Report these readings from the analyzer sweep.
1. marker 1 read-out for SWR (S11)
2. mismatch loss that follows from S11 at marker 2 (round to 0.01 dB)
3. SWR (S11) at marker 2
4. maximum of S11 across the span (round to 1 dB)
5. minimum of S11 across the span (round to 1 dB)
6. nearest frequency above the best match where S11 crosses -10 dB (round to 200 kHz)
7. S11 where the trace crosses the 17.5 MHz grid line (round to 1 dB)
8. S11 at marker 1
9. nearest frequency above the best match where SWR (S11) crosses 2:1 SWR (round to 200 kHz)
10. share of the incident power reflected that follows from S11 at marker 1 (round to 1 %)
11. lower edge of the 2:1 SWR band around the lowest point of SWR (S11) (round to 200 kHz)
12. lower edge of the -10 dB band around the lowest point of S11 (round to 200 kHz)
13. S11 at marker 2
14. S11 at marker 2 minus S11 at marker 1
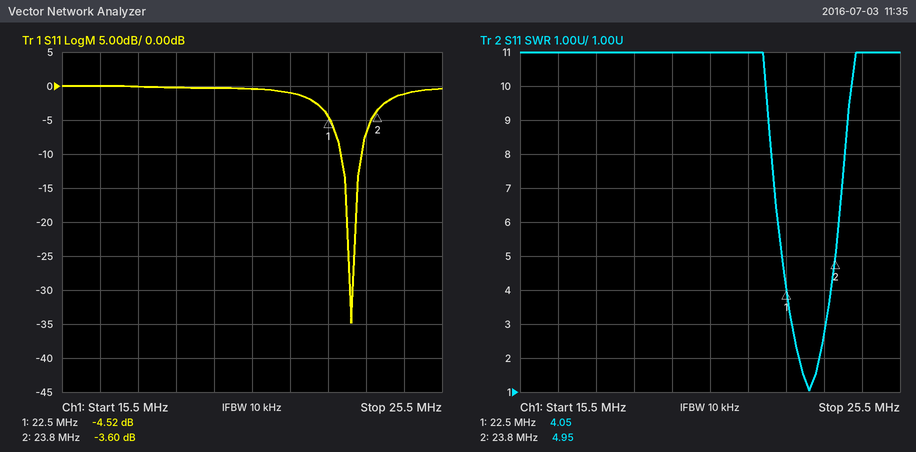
4.05
2.49 dB
4.95
0 dB
-35 dB
23.4 MHz
0 dB
-4.52 dB
23.4 MHz
35 %
22.8 MHz
22.8 MHz
-3.60 dB
0.92 dB
